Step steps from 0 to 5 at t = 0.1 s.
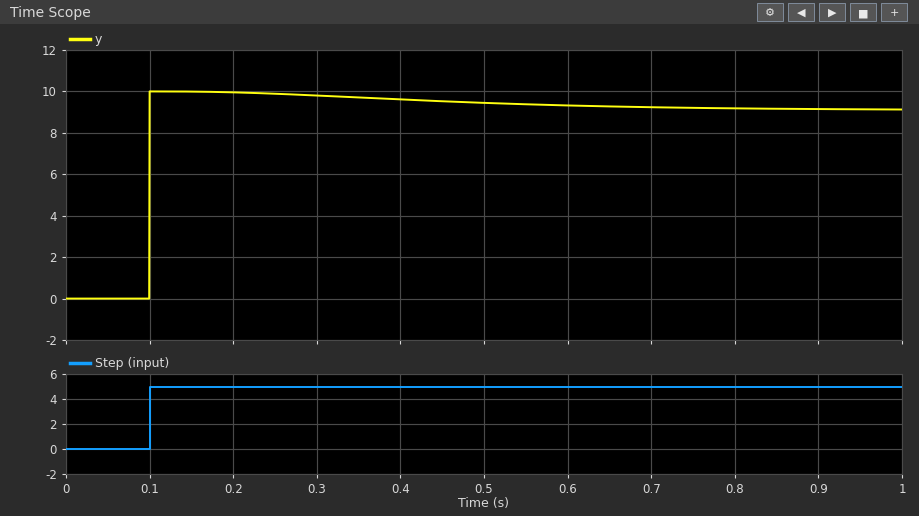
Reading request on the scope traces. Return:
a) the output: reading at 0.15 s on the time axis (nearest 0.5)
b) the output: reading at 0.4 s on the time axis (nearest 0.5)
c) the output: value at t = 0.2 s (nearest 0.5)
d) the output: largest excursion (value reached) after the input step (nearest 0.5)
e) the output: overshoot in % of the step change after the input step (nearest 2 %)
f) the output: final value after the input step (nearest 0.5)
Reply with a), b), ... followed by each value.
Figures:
a) 10.0
b) 9.5
c) 10.0
d) 10.0
e) 10 %
f) 9.0
